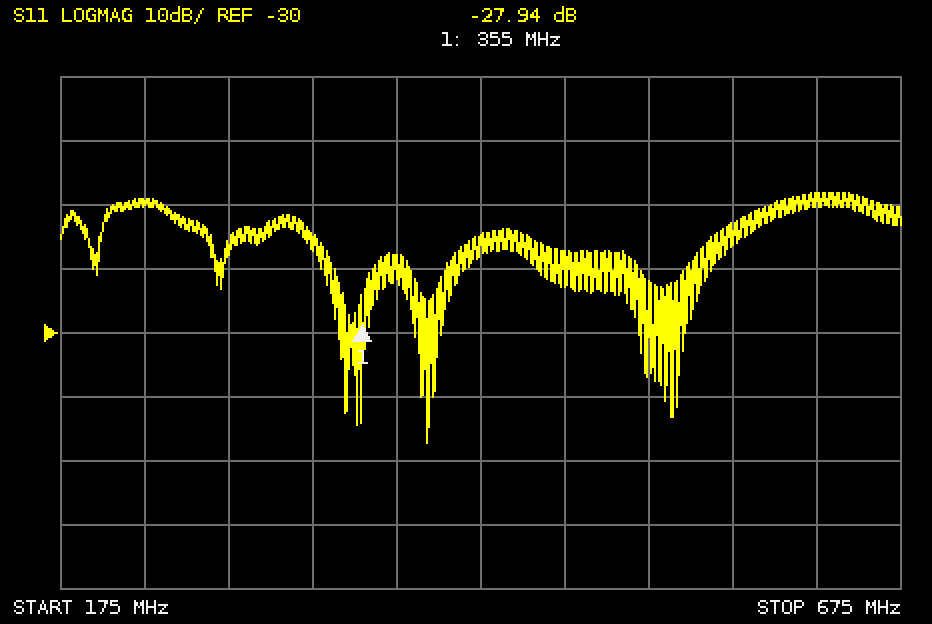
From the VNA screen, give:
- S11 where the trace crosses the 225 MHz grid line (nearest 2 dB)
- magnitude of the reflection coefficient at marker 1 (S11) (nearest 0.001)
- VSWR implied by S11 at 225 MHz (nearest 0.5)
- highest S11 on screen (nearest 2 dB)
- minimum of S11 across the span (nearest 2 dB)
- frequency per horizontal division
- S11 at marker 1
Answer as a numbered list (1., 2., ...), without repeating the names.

1. -10 dB
2. 0.040
3. 2.0
4. -8 dB
5. -48 dB
6. 50 MHz
7. -27.94 dB
